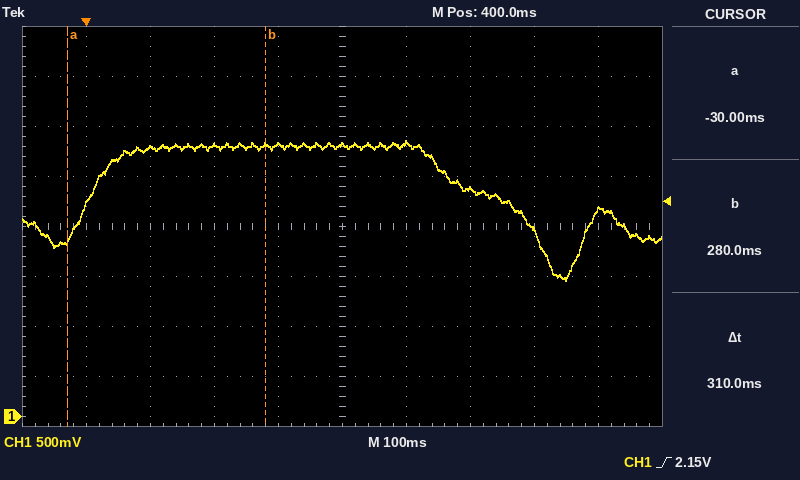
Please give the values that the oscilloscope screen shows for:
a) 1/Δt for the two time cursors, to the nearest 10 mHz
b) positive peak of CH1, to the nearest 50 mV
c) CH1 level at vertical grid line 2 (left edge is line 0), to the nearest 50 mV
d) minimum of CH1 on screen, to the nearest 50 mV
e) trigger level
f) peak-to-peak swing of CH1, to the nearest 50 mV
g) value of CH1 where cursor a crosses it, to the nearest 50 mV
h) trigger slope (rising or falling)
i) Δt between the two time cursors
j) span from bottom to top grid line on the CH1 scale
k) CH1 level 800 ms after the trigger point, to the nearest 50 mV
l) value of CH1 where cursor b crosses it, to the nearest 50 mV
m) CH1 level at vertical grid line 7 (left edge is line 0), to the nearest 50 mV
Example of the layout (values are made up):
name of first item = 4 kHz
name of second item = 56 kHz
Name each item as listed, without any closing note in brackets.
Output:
1/Δt for the two time cursors, to the nearest 10 mHz = 3.23 Hz
positive peak of CH1, to the nearest 50 mV = 2.75 V
CH1 level at vertical grid line 2 (left edge is line 0), to the nearest 50 mV = 2.70 V
minimum of CH1 on screen, to the nearest 50 mV = 1.35 V
trigger level = 2.15 V
peak-to-peak swing of CH1, to the nearest 50 mV = 1.40 V
value of CH1 where cursor a crosses it, to the nearest 50 mV = 1.75 V
trigger slope = rising
Δt between the two time cursors = 310 ms
span from bottom to top grid line on the CH1 scale = 4 V
CH1 level 800 ms after the trigger point, to the nearest 50 mV = 2.05 V
value of CH1 where cursor b crosses it, to the nearest 50 mV = 2.70 V
CH1 level at vertical grid line 7 (left edge is line 0), to the nearest 50 mV = 2.30 V
